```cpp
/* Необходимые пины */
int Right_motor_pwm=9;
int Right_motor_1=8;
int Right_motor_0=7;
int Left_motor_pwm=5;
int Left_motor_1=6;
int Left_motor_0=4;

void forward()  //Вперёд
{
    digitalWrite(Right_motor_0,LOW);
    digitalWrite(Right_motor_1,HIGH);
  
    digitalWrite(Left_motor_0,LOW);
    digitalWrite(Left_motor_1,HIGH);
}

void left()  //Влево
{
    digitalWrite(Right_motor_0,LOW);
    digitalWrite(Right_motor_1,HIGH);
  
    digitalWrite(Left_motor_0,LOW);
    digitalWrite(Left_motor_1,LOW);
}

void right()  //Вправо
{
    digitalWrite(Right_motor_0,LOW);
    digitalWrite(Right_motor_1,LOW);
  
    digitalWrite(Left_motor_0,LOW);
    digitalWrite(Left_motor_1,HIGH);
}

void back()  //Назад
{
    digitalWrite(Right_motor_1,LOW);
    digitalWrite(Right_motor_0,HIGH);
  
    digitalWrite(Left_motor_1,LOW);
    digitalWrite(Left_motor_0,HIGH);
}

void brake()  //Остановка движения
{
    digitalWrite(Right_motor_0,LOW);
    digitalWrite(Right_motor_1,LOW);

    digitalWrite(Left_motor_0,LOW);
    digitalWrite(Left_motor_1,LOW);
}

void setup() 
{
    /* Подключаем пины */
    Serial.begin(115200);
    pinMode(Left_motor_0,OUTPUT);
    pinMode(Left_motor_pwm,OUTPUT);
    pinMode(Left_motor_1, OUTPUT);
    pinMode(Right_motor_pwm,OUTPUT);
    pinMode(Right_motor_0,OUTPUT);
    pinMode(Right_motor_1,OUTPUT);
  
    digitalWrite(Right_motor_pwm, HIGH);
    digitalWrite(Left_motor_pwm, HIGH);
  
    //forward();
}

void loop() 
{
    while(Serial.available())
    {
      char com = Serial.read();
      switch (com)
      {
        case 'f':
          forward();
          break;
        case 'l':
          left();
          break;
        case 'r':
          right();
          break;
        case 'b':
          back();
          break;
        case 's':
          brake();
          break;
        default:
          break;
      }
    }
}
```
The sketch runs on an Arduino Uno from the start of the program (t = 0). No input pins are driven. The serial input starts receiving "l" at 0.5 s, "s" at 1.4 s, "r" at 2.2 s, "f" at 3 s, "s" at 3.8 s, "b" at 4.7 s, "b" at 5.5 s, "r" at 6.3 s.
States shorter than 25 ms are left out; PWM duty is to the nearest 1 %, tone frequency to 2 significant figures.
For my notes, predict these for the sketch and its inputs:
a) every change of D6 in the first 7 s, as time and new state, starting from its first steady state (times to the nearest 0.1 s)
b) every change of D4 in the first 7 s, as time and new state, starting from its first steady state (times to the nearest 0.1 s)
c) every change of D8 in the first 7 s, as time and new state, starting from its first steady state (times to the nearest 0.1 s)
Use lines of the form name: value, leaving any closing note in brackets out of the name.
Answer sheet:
every change of D6 in the first 7 s, as time and new state, starting from its first steady state: 0 s low; 2.2 s high; 3.8 s low; 6.3 s high
every change of D4 in the first 7 s, as time and new state, starting from its first steady state: 0 s low; 4.7 s high; 6.3 s low
every change of D8 in the first 7 s, as time and new state, starting from its first steady state: 0 s low; 0.5 s high; 1.4 s low; 3 s high; 3.8 s low
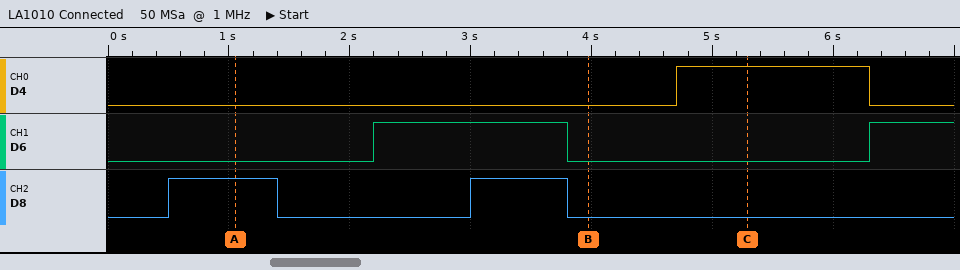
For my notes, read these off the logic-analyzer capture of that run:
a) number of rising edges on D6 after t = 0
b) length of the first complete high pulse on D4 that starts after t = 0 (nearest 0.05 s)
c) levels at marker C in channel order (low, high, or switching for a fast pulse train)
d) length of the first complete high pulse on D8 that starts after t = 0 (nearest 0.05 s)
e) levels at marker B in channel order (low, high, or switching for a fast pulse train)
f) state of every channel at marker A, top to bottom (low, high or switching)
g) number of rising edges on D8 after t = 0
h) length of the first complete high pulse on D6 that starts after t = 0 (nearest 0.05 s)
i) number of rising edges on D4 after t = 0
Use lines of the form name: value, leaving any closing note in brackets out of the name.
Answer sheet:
number of rising edges on D6 after t = 0: 2
length of the first complete high pulse on D4 that starts after t = 0: 1.60 s
levels at marker C in channel order: D4 high, D6 low, D8 low
length of the first complete high pulse on D8 that starts after t = 0: 0.90 s
levels at marker B in channel order: D4 low, D6 low, D8 low
state of every channel at marker A, top to bottom: D4 low, D6 low, D8 high
number of rising edges on D8 after t = 0: 2
length of the first complete high pulse on D6 that starts after t = 0: 1.60 s
number of rising edges on D4 after t = 0: 1
